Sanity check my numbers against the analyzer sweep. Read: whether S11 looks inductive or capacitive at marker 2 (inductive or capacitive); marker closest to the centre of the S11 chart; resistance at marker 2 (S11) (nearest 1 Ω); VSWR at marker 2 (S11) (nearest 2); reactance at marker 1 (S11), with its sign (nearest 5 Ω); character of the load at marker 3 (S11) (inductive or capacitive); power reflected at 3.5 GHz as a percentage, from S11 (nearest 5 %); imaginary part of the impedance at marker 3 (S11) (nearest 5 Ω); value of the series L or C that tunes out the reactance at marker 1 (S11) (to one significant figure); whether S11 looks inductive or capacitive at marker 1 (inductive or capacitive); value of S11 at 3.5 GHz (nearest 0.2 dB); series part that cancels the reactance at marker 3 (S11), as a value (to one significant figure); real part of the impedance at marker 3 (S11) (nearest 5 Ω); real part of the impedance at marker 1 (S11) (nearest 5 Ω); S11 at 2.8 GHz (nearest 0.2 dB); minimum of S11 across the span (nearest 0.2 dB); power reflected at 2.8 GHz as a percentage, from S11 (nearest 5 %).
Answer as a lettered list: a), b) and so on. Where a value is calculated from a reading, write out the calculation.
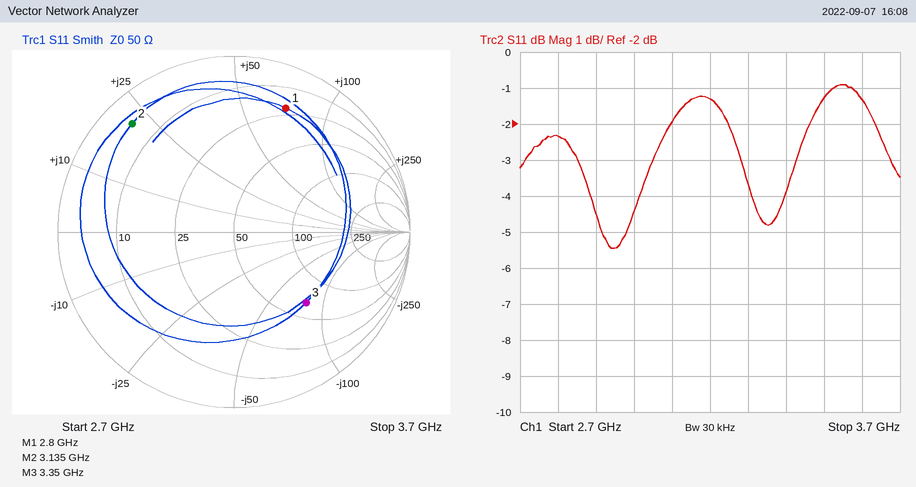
a) inductive
b) marker 3
c) 5 Ω
d) 12
e) +70 Ω
f) capacitive
g) 10^(-1.2/10) ≈ 75.9 %, so 75 % to the nearest 5 %
h) -80 Ω
i) C = 1/(2π × 2.8 GHz × 70 Ω) ≈ 812 fF, so 800 fF to one significant figure
j) inductive
k) -1.2 dB
l) L = 80 Ω/(2π × 3.35 GHz) ≈ 4 nH
m) 65 Ω
n) 20 Ω
o) -2.4 dB
p) -5.4 dB
q) 10^(-2.4/10) ≈ 57.5 %, so 60 % to the nearest 5 %
